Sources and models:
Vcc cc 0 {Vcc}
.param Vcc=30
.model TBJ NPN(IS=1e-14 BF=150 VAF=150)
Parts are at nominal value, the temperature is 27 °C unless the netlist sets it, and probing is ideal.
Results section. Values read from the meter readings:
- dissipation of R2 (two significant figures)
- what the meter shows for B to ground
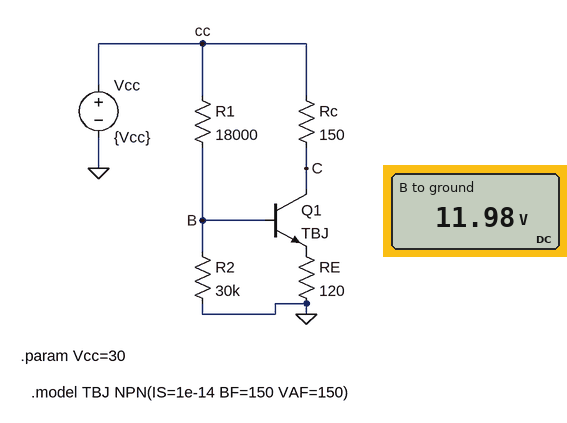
4.8 mW
11.98 V
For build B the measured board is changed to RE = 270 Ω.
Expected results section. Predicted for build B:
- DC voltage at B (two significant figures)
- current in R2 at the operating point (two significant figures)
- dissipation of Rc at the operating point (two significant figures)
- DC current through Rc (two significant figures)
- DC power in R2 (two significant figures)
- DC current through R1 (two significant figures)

15 V
500 µA
410 mW
52 mA
7.5 mW
830 µA
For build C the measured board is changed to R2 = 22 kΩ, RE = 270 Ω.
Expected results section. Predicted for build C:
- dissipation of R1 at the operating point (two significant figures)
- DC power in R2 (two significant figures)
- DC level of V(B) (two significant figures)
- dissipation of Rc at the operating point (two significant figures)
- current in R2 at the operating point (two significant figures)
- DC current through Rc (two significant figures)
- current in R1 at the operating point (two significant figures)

15 mW
8.4 mW
14 V
330 mW
620 µA
47 mA
910 µA
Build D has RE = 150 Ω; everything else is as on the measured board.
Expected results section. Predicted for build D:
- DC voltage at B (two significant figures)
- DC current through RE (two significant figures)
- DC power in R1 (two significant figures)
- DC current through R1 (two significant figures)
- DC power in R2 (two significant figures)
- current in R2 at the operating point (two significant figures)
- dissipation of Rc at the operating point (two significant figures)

13 V
81 mA
16 mW
950 µA
5.6 mW
430 µA
970 mW
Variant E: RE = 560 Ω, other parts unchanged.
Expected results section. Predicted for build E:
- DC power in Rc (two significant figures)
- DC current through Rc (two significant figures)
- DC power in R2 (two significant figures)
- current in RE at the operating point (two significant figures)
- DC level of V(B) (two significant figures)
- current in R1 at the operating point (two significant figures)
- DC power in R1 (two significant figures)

120 mW
28 mA
9.3 mW
29 mA
17 V
740 µA
9.8 mW
